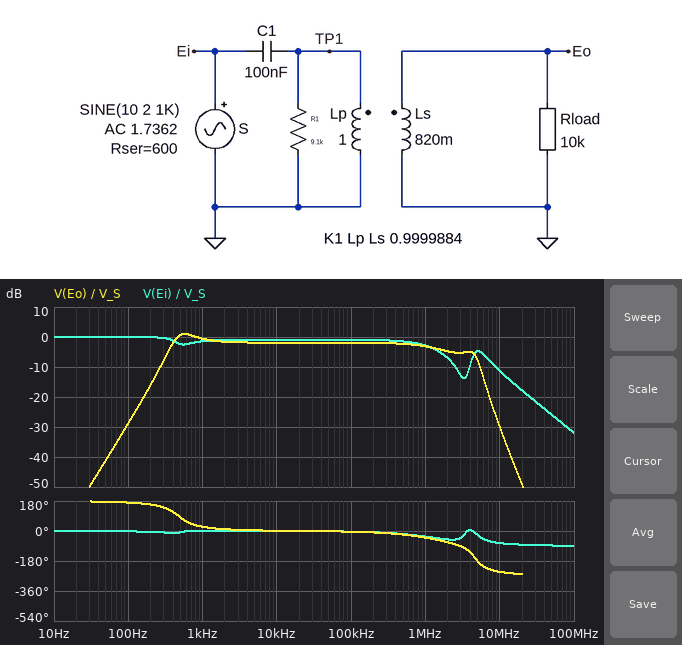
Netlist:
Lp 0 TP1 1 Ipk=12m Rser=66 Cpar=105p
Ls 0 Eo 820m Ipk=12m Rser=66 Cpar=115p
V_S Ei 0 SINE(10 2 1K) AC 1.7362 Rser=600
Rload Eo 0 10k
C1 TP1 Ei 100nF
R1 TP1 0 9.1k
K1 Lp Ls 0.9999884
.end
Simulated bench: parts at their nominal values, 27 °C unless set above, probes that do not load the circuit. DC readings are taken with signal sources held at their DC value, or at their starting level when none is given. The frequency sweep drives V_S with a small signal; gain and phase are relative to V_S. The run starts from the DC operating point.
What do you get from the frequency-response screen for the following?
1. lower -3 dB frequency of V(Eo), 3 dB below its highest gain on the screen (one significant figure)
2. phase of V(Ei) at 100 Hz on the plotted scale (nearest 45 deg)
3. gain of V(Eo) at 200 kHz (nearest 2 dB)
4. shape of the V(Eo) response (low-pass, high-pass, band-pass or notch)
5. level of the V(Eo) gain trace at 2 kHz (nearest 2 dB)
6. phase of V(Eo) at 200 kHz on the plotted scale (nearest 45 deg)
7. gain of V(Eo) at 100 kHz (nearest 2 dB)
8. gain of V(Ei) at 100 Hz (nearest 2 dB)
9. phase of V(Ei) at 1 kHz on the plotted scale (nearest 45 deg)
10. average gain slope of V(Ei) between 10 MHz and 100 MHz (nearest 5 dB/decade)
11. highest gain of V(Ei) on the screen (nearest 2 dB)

400 Hz
0 deg
-2 dB
band-pass
-2 dB
0 deg
-2 dB
0 dB
0 deg
-20 dB/decade
0 dB
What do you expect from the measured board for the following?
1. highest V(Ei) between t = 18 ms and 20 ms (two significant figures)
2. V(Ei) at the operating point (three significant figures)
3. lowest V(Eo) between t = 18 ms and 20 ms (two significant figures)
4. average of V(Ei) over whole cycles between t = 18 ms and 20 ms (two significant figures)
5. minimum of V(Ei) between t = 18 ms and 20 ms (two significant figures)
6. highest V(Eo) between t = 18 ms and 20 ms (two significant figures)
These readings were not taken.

12 V
10.0 V
-1.9 V
10 V
8.3 V
1.9 V
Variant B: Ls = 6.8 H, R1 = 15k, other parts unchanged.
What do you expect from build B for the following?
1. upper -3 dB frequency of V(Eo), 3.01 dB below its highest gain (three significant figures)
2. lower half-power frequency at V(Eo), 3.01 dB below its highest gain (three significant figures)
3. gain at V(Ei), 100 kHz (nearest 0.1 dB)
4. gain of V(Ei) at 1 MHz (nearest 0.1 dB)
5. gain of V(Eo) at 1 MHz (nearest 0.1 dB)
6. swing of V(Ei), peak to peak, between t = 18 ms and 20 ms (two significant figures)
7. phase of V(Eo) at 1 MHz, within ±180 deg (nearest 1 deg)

440 kHz
681 Hz
-3.3 dB
-15.9 dB
-2.8 dB
3.2 V
-81 deg
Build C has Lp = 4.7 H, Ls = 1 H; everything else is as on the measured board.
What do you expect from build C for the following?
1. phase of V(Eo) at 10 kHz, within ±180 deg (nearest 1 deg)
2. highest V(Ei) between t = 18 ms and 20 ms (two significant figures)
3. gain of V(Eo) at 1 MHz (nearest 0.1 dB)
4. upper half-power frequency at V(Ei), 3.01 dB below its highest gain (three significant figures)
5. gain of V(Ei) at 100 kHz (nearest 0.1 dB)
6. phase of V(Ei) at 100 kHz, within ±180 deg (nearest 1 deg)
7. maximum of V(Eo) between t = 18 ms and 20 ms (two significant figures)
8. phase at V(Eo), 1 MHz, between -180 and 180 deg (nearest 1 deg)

1 deg
12 V
-7.4 dB
1.67 MHz
-0.7 dB
-3 deg
870 mV
-29 deg
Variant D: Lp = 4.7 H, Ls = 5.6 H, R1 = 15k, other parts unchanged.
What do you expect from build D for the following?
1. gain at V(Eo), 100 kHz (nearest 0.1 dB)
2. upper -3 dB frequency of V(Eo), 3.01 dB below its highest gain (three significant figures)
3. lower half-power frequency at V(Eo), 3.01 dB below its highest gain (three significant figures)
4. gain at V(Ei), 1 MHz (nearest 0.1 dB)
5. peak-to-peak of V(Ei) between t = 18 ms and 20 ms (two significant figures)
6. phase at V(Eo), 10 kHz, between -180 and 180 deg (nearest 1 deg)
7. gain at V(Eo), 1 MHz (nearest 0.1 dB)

-0.3 dB
1.83 MHz
246 Hz
-6.5 dB
3.6 V
1 deg
0.9 dB
